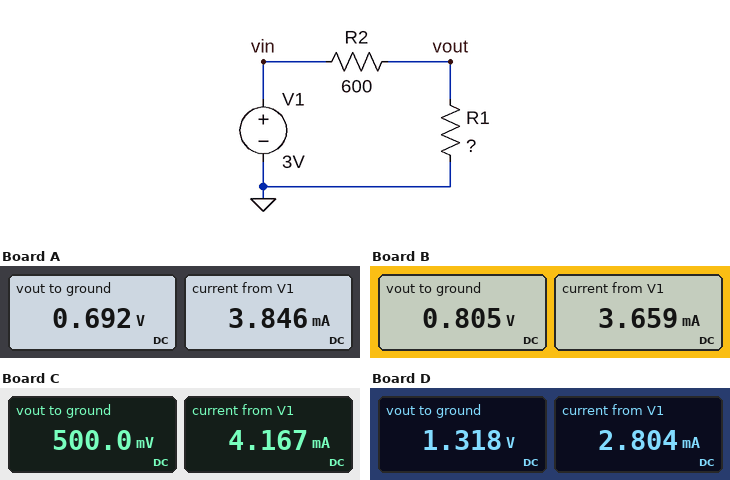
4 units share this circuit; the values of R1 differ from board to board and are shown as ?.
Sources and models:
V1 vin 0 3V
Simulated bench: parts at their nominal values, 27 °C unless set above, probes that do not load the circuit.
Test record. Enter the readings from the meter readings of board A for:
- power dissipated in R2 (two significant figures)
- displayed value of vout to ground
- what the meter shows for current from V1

8.9 mW
0.692 V
3.846 mA
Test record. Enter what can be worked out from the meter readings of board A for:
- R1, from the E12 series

180 Ω
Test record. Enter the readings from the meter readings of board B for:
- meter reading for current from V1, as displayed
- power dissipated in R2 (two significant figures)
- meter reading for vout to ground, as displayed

3.659 mA
8.0 mW
0.805 V
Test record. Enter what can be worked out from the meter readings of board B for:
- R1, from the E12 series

220 Ω
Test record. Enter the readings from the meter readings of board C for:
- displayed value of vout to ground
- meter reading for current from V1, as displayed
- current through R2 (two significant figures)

500.0 mV
4.167 mA
4.2 mA
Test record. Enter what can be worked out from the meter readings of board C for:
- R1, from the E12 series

120 Ω
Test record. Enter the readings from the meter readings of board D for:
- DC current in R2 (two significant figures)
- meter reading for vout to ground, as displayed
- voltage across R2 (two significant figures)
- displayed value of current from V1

2.8 mA
1.318 V
1.7 V
2.804 mA
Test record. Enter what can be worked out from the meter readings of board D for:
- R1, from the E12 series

470 Ω
